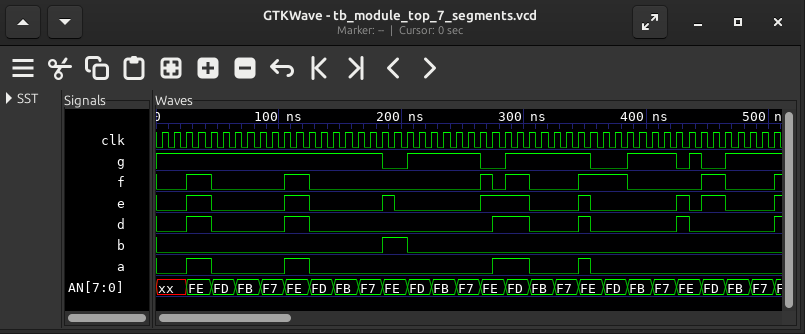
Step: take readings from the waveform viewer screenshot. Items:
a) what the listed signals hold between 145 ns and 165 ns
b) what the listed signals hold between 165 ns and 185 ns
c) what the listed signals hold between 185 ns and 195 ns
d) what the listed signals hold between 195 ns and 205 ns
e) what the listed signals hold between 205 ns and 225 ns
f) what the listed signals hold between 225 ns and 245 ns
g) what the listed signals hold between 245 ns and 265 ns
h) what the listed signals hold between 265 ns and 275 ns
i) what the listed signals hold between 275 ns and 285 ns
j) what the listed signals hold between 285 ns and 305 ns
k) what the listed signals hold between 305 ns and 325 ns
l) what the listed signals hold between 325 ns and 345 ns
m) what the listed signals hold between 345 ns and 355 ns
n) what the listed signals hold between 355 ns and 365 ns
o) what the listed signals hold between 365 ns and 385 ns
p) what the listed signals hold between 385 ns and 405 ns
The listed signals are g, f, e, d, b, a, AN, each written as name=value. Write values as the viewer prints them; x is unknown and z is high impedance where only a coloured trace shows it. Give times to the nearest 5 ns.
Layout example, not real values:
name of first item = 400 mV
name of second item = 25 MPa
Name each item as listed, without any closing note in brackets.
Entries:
what the listed signals hold between 145 ns and 165 ns = g=1, f=0, e=0, d=0, b=0, a=0, AN=FB
what the listed signals hold between 165 ns and 185 ns = g=1, f=0, e=0, d=0, b=0, a=0, AN=F7
what the listed signals hold between 185 ns and 195 ns = g=0, f=0, e=1, d=0, b=1, a=0, AN=FE
what the listed signals hold between 195 ns and 205 ns = g=0, f=0, e=0, d=0, b=1, a=0, AN=FE
what the listed signals hold between 205 ns and 225 ns = g=1, f=0, e=0, d=0, b=0, a=0, AN=FD
what the listed signals hold between 225 ns and 245 ns = g=1, f=0, e=0, d=0, b=0, a=0, AN=FB
what the listed signals hold between 245 ns and 265 ns = g=1, f=0, e=0, d=0, b=0, a=0, AN=F7
what the listed signals hold between 265 ns and 275 ns = g=0, f=1, e=1, d=0, b=0, a=0, AN=FE
what the listed signals hold between 275 ns and 285 ns = g=0, f=0, e=1, d=1, b=0, a=1, AN=FE
what the listed signals hold between 285 ns and 305 ns = g=1, f=1, e=1, d=1, b=0, a=1, AN=FD
what the listed signals hold between 305 ns and 325 ns = g=1, f=0, e=0, d=0, b=0, a=0, AN=FB
what the listed signals hold between 325 ns and 345 ns = g=1, f=0, e=0, d=0, b=0, a=0, AN=F7
what the listed signals hold between 345 ns and 355 ns = g=1, f=1, e=1, d=1, b=0, a=1, AN=FE
what the listed signals hold between 355 ns and 365 ns = g=0, f=1, e=0, d=0, b=0, a=0, AN=FE
what the listed signals hold between 365 ns and 385 ns = g=0, f=1, e=0, d=0, b=0, a=0, AN=FD
what the listed signals hold between 385 ns and 405 ns = g=1, f=0, e=0, d=0, b=0, a=0, AN=FB
